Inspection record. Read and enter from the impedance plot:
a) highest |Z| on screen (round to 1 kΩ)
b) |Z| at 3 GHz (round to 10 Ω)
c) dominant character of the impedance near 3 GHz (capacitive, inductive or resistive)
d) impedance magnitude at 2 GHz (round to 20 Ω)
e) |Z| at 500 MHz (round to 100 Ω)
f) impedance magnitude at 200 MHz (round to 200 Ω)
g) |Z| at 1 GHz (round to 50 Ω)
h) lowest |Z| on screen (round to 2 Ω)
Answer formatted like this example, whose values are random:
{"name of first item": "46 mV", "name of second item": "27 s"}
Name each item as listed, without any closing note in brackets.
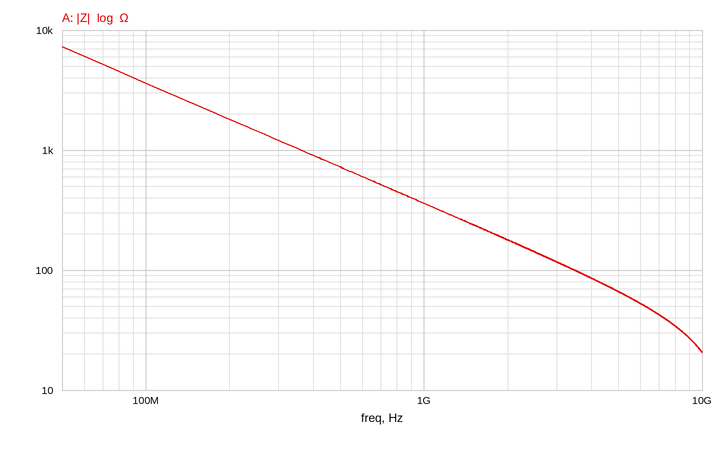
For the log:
{"highest |Z| on screen": "7 kΩ", "|Z| at 3 GHz": "120 Ω", "dominant character of the impedance near 3 GHz": "capacitive", "impedance magnitude at 2 GHz": "180 Ω", "|Z| at 500 MHz": "700 Ω", "impedance magnitude at 200 MHz": "1.8 kΩ", "|Z| at 1 GHz": "350 Ω", "lowest |Z| on screen": "20 Ω"}
